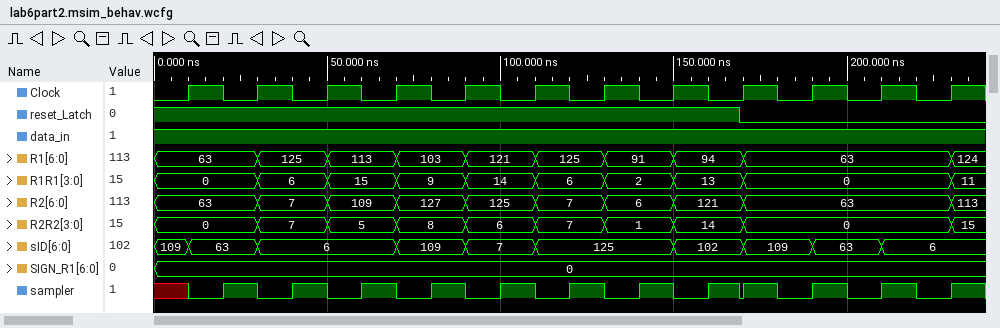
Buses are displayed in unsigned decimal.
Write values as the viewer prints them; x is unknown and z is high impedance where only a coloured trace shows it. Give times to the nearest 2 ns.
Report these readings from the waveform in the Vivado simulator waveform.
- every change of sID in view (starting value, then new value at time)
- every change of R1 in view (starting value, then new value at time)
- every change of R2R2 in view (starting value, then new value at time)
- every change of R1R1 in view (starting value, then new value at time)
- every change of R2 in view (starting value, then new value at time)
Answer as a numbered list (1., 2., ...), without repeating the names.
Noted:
1. 109, 63 at 10 ns, 6 at 30 ns, 109 at 70 ns, 7 at 90 ns, 125 at 110 ns, 102 at 150 ns, 109 at 170 ns, 63 at 190 ns, 6 at 210 ns
2. 63, 125 at 30 ns, 113 at 50 ns, 103 at 70 ns, 121 at 90 ns, 125 at 110 ns, 91 at 130 ns, 94 at 150 ns, 63 at 170 ns, 124 at 230 ns
3. 0, 7 at 30 ns, 5 at 50 ns, 8 at 70 ns, 6 at 90 ns, 7 at 110 ns, 1 at 130 ns, 14 at 150 ns, 0 at 170 ns, 15 at 230 ns
4. 0, 6 at 30 ns, 15 at 50 ns, 9 at 70 ns, 14 at 90 ns, 6 at 110 ns, 2 at 130 ns, 13 at 150 ns, 0 at 170 ns, 11 at 230 ns
5. 63, 7 at 30 ns, 109 at 50 ns, 127 at 70 ns, 125 at 90 ns, 7 at 110 ns, 6 at 130 ns, 121 at 150 ns, 63 at 170 ns, 113 at 230 ns
